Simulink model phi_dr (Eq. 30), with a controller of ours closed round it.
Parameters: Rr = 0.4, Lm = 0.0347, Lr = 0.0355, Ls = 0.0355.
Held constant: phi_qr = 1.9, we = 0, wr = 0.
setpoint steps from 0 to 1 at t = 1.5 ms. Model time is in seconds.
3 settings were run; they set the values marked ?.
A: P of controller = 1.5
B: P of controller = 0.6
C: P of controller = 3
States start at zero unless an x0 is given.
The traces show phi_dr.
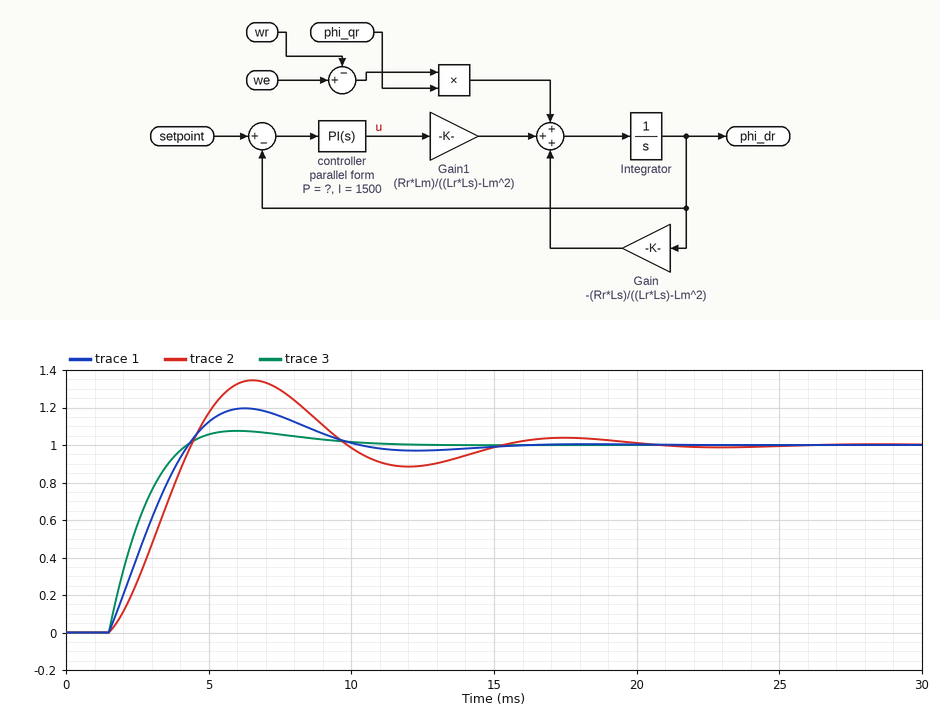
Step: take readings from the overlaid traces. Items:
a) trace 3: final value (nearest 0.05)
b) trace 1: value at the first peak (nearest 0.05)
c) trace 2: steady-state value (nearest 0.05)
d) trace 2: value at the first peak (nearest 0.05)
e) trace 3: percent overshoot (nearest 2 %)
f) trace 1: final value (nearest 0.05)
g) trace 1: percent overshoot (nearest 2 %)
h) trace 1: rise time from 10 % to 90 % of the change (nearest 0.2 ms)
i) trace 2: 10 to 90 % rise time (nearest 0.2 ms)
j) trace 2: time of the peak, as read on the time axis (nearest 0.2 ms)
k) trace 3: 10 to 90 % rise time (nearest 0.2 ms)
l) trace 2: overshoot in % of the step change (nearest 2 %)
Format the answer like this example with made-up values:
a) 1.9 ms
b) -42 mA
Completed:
a) 1.00
b) 1.20
c) 1.00
d) 1.35
e) 8 %
f) 1.00
g) 20 %
h) 2.2 ms
i) 2.2 ms
j) 6.6 ms
k) 2.0 ms
l) 34 %
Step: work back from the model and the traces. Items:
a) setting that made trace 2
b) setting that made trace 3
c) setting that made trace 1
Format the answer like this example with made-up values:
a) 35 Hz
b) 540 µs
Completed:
a) B
b) C
c) A
